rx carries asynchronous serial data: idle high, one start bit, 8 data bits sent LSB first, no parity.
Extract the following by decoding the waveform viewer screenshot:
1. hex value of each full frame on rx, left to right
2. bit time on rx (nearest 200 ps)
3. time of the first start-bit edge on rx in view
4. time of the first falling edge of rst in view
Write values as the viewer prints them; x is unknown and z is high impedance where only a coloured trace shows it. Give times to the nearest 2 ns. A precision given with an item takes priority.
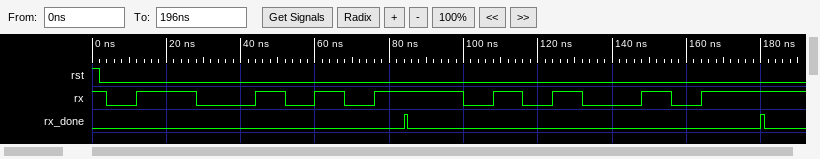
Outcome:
53, A5
8000 ps
4 ns
2 ns
